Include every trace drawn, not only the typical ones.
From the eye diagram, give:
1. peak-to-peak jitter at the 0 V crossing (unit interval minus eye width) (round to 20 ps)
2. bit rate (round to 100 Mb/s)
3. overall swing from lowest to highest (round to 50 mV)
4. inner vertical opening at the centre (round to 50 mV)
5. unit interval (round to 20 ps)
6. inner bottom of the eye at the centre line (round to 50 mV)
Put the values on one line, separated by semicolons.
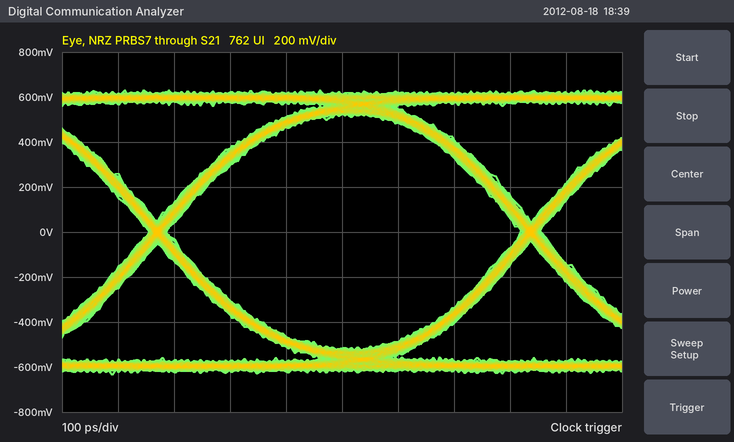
40 ps; 1.5 Gb/s; 1.25 V; 1.05 V; 660 ps; -500 mV
